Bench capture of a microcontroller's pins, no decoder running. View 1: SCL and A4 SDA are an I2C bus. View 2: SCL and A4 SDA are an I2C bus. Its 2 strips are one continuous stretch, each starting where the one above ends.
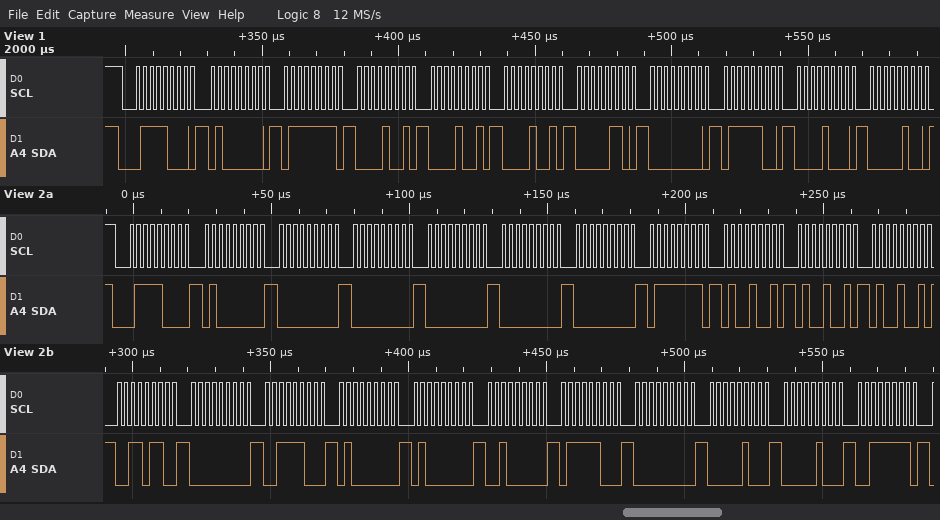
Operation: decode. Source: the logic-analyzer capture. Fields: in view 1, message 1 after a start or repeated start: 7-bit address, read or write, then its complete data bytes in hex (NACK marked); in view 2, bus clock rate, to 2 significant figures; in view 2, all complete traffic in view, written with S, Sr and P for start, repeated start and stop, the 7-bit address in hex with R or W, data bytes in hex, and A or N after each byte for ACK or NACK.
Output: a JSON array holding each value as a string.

["0x3C write: 40 7F 09 09 09 06 00 7C 08 04", "400 kHz", "S 3CW A 40 A 00 A 00 A 00 A 00 A 00 A 7F A 49 A 49 A 49 A 36 A 00 A 3C A 40 A 40 A 20 A 7C A 00 A 04 A 04 A 3F A"]
